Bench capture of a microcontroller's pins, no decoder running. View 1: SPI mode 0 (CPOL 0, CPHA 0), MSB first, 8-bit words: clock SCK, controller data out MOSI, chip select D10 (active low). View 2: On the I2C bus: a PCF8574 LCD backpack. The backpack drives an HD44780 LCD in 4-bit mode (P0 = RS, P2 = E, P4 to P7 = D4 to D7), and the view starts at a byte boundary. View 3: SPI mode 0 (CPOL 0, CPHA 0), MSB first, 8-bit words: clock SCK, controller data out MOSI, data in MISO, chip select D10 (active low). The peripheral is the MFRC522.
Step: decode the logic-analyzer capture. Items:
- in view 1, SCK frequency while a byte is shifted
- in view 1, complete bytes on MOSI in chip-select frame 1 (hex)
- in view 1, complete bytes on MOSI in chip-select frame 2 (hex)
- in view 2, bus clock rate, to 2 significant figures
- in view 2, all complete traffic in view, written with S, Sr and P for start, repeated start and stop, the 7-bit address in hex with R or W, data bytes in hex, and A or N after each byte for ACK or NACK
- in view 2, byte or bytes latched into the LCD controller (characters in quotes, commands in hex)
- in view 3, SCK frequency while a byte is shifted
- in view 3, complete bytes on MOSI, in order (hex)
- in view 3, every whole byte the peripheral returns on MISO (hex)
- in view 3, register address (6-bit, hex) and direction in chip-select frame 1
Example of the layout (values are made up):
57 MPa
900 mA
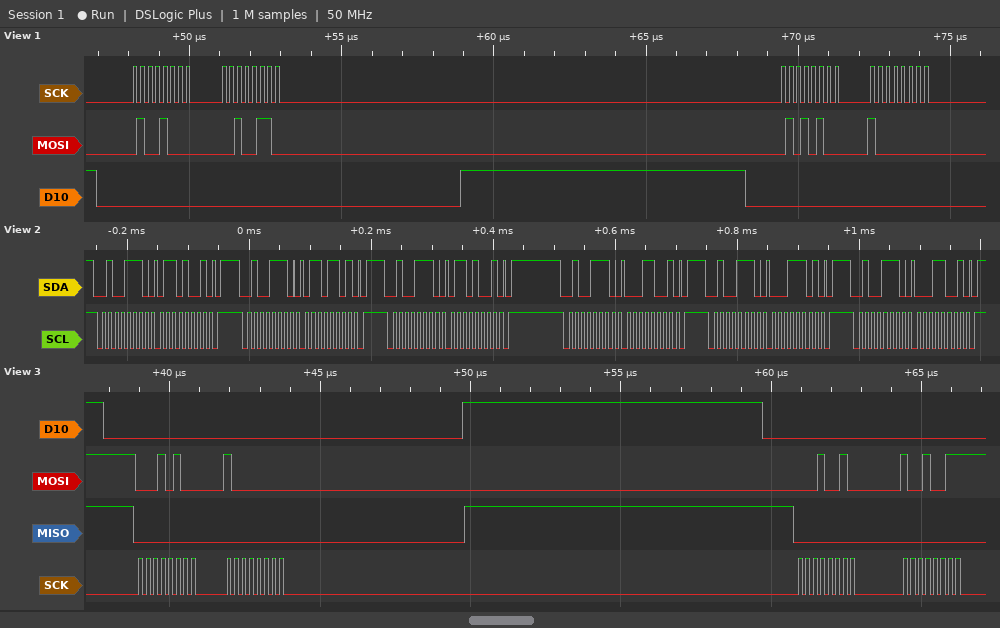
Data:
4 MHz
48 26
54 80
100 kHz
S 27W A 69 A P S 27W A 6D A P S 27W A 69 A P S 27W A 19 A P S 27W A 1D A P S 27W A 19 A P
'a'
4 MHz
0x14 0x80 0x12 0x93
0x00 0x00 0x00 0x00
0x0A write
